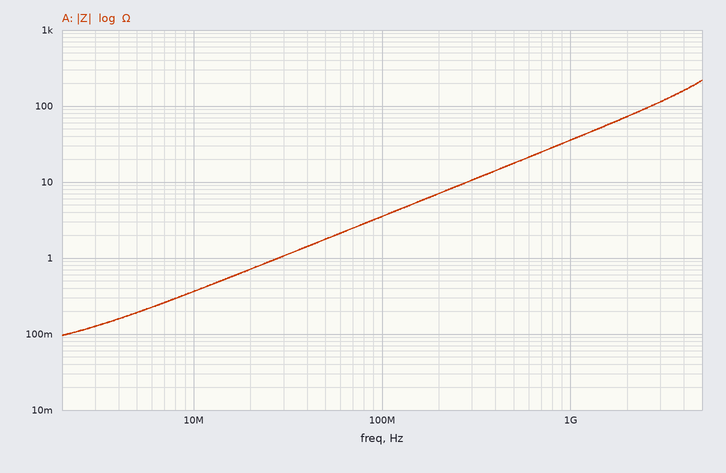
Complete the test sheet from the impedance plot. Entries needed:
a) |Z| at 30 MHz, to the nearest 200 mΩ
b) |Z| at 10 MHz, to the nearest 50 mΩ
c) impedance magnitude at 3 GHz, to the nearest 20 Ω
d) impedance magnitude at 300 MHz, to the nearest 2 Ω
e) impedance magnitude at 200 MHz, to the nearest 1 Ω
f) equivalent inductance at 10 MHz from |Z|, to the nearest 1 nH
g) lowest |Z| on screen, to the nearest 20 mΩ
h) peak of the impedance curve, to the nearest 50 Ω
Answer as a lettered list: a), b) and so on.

a) 1.0 Ω
b) 350 mΩ
c) 120 Ω
d) 10 Ω
e) 7 Ω
f) 6 nH
g) 100 mΩ
h) 200 Ω
